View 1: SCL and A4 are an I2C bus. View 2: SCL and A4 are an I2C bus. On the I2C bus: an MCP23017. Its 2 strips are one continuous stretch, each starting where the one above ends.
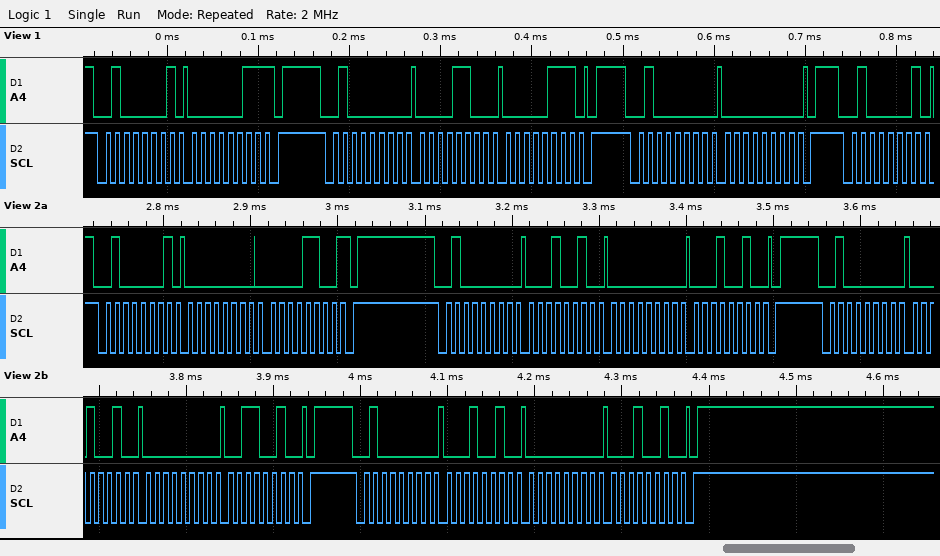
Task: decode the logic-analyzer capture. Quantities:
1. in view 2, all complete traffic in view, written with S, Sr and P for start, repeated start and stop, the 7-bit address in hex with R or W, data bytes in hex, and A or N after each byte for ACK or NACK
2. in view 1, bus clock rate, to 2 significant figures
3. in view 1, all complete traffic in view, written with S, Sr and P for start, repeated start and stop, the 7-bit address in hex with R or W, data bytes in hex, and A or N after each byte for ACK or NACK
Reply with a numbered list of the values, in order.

1. S 20R A 00 A 0C N P S 20W A 12 A 00 A 12 A P S 20W A 12 A 00 A 32 A P S 20W A 12 A 00 A 12 A P
2. 100 kHz
3. S 20R A 03 N P S 20W A 0C A 07 A P S 20W A 00 A P S 20R A
